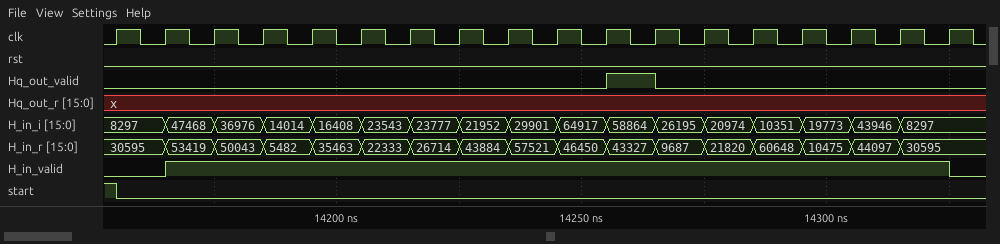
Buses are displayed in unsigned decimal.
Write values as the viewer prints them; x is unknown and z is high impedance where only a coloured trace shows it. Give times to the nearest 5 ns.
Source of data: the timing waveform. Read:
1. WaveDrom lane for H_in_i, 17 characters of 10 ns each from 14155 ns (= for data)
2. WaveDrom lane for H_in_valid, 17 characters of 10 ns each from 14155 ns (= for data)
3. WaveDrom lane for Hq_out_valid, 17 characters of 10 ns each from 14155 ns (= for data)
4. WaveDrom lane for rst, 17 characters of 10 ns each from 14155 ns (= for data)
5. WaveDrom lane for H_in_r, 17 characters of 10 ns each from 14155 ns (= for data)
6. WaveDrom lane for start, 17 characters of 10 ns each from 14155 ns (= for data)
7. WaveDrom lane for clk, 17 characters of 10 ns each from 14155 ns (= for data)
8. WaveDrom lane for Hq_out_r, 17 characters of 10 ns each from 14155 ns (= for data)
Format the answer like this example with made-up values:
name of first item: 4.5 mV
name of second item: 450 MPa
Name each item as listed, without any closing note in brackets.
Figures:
WaveDrom lane for H_in_i, 17 characters of 10 ns each from 14155 ns: {name: 'H_in_i', wave: '=================', data: '8297 47468 36976 14014 16408 23543 23777 21952 29901 64917 58864 26195 20974 10351 19773 43946 8297'}
WaveDrom lane for H_in_valid, 17 characters of 10 ns each from 14155 ns: {name: 'H_in_valid', wave: '01...............'}
WaveDrom lane for Hq_out_valid, 17 characters of 10 ns each from 14155 ns: {name: 'Hq_out_valid', wave: '0.........10.....'}
WaveDrom lane for rst, 17 characters of 10 ns each from 14155 ns: {name: 'rst', wave: '0................'}
WaveDrom lane for H_in_r, 17 characters of 10 ns each from 14155 ns: {name: 'H_in_r', wave: '=================', data: '30595 53419 50043 5482 35463 22333 26714 43884 57521 46450 43327 9687 21820 60648 10475 44097 30595'}
WaveDrom lane for start, 17 characters of 10 ns each from 14155 ns: {name: 'start', wave: '0................'}
WaveDrom lane for clk, 17 characters of 10 ns each from 14155 ns: {name: 'clk', wave: 'p................'}
WaveDrom lane for Hq_out_r, 17 characters of 10 ns each from 14155 ns: {name: 'Hq_out_r', wave: 'x................'}
